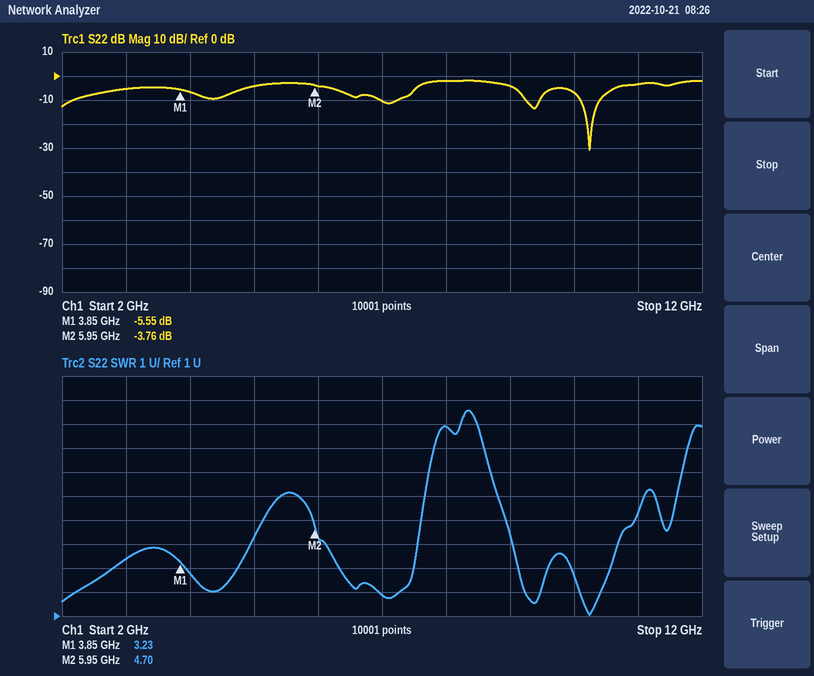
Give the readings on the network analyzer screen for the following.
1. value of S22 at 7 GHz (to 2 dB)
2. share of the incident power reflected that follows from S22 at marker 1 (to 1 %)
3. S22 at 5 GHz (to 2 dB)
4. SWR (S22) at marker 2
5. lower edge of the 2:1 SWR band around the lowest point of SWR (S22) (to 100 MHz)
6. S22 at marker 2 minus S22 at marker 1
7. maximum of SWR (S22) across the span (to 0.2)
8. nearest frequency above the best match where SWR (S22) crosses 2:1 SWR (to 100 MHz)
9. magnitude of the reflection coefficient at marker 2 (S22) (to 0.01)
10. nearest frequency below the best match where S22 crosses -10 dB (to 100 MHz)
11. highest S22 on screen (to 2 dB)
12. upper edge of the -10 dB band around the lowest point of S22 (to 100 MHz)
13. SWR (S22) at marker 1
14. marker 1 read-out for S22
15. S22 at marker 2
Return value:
-10 dB
28 %
-4 dB
4.70
10.1 GHz
1.79 dB
9.6
10.4 GHz
0.65
10.1 GHz
-2 dB
10.4 GHz
3.23
-5.55 dB
-3.76 dB
